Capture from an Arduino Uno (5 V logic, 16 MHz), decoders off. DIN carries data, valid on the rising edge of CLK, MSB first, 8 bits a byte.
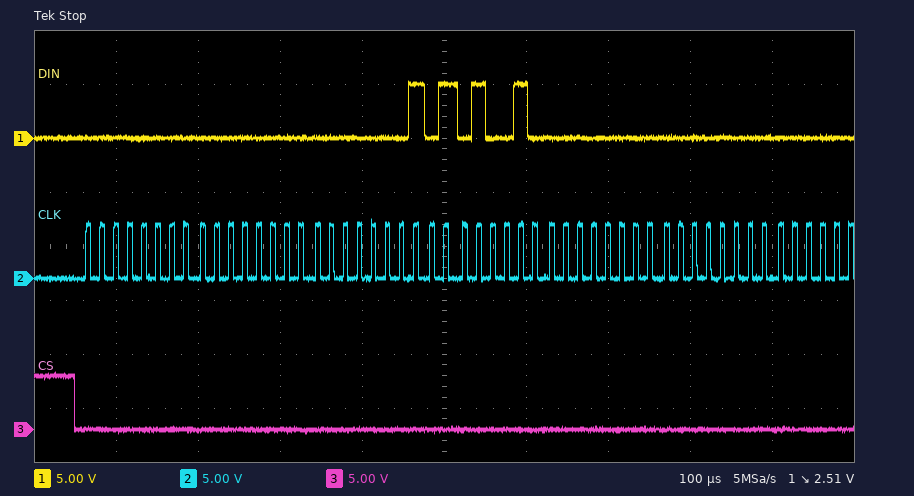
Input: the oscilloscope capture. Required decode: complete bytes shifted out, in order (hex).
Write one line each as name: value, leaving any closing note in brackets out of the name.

complete bytes shifted out, in order: 00 00 01 52 00 00
